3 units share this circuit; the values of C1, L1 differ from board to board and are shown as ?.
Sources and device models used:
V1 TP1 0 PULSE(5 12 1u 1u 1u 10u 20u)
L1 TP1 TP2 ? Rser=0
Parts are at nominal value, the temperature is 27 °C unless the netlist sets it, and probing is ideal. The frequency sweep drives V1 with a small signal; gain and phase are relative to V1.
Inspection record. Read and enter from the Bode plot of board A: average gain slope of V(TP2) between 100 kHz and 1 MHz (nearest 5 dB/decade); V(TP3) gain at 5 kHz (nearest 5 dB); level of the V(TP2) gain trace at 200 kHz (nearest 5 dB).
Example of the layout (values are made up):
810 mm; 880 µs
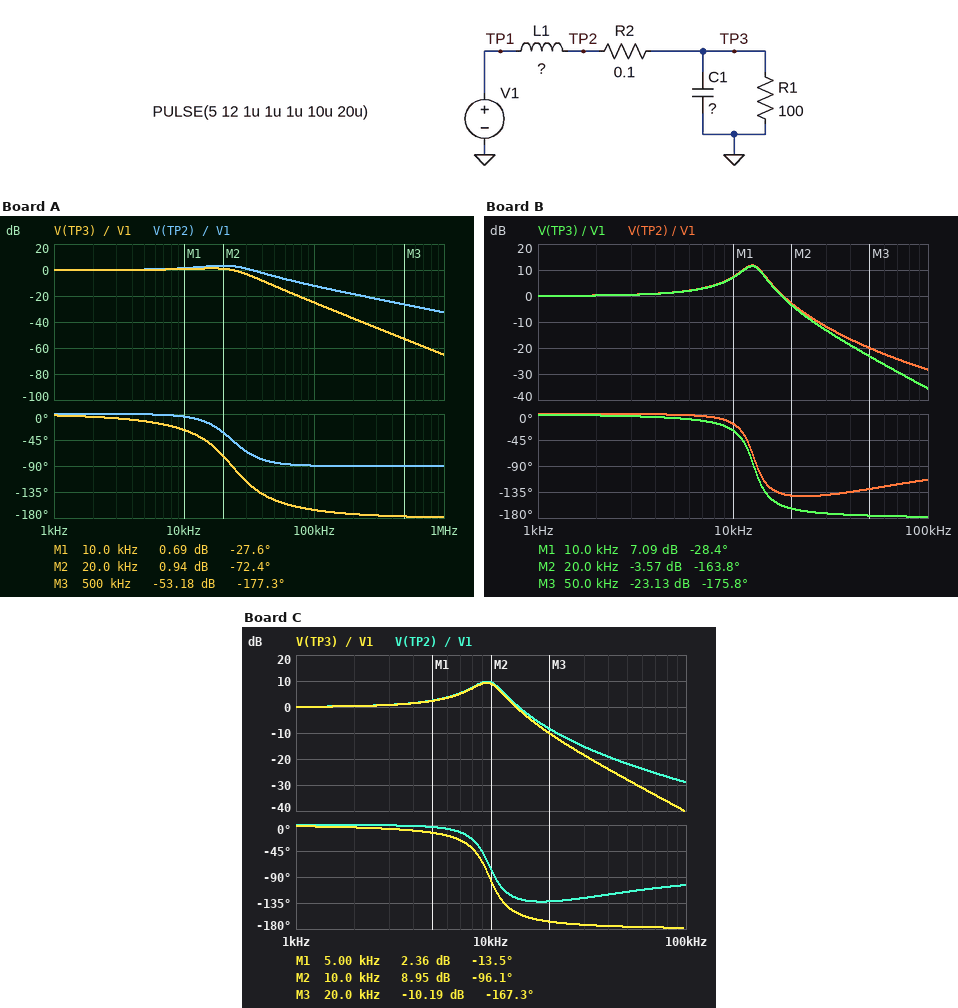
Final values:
-20 dB/decade; 0 dB; -20 dB
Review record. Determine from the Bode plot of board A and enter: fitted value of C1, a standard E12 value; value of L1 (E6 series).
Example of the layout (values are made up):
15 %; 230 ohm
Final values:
68 µF; 680 nH
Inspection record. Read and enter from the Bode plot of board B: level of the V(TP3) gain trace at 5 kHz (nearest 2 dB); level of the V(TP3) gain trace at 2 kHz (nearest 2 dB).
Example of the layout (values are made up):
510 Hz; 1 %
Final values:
2 dB; 0 dB
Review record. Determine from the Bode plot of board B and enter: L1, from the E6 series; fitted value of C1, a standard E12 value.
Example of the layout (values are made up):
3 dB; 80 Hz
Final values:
4.7 µH; 33 µF
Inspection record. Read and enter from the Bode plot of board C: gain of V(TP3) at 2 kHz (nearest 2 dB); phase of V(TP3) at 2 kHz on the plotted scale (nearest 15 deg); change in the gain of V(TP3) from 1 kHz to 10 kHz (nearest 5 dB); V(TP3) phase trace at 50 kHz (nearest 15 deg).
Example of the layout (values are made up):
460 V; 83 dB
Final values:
0 dB; 0 deg; 10 dB; -180 deg
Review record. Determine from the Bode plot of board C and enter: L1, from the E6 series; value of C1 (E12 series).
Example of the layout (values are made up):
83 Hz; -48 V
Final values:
4.7 µH; 56 µF
